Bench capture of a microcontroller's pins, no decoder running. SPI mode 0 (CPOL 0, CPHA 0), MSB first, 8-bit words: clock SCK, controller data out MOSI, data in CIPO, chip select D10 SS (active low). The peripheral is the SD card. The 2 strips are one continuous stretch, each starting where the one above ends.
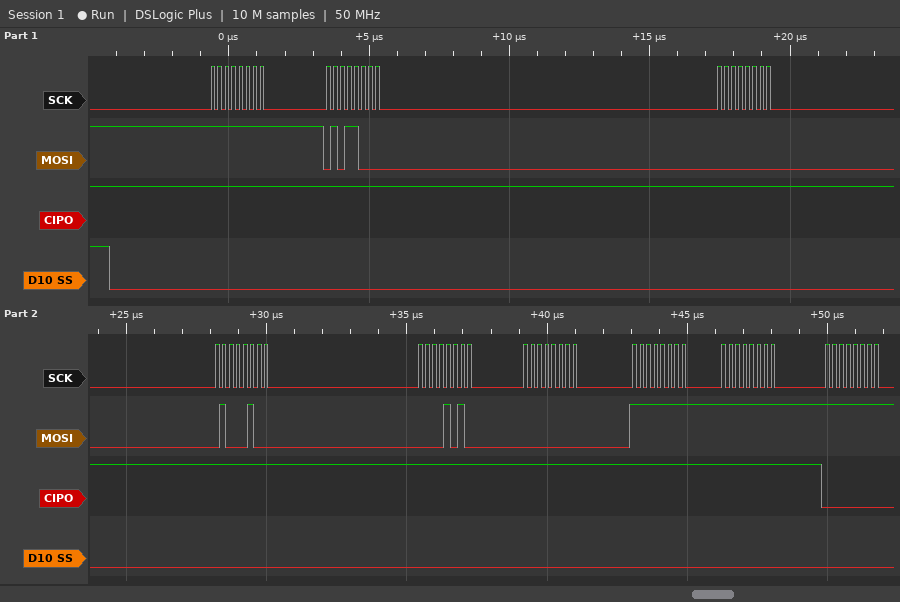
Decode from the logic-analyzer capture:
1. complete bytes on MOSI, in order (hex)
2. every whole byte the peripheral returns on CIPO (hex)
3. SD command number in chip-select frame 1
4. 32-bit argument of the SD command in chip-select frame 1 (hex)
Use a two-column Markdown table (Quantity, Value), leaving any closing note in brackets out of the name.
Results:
| Quantity | Value |
|---|---|
| complete bytes on MOSI, in order | FF 58 00 44 0A 00 FF FF FF |
| every whole byte the peripheral returns on CIPO | FF FF FF FF FF FF FF FF 00 |
| SD command number in chip-select frame 1 | CMD24 |
| 32-bit argument of the SD command in chip-select frame 1 | 0x00440A00 |
